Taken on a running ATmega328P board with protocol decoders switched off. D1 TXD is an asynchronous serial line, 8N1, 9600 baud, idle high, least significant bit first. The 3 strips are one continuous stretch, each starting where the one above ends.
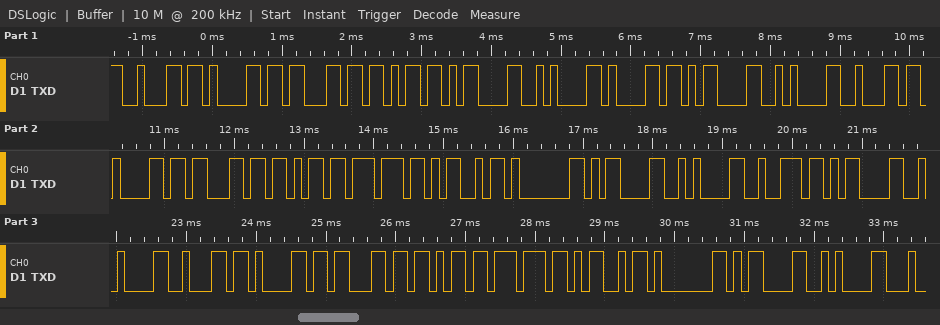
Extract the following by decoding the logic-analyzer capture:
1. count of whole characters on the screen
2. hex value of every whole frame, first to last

30
62 61 63 6B 0D 0A 61 0D 0A 62 61 63 6B 77 4D 01 0D 0A 72 0D 0A 62 61 63 6B 77 4D 01 0D 0A
